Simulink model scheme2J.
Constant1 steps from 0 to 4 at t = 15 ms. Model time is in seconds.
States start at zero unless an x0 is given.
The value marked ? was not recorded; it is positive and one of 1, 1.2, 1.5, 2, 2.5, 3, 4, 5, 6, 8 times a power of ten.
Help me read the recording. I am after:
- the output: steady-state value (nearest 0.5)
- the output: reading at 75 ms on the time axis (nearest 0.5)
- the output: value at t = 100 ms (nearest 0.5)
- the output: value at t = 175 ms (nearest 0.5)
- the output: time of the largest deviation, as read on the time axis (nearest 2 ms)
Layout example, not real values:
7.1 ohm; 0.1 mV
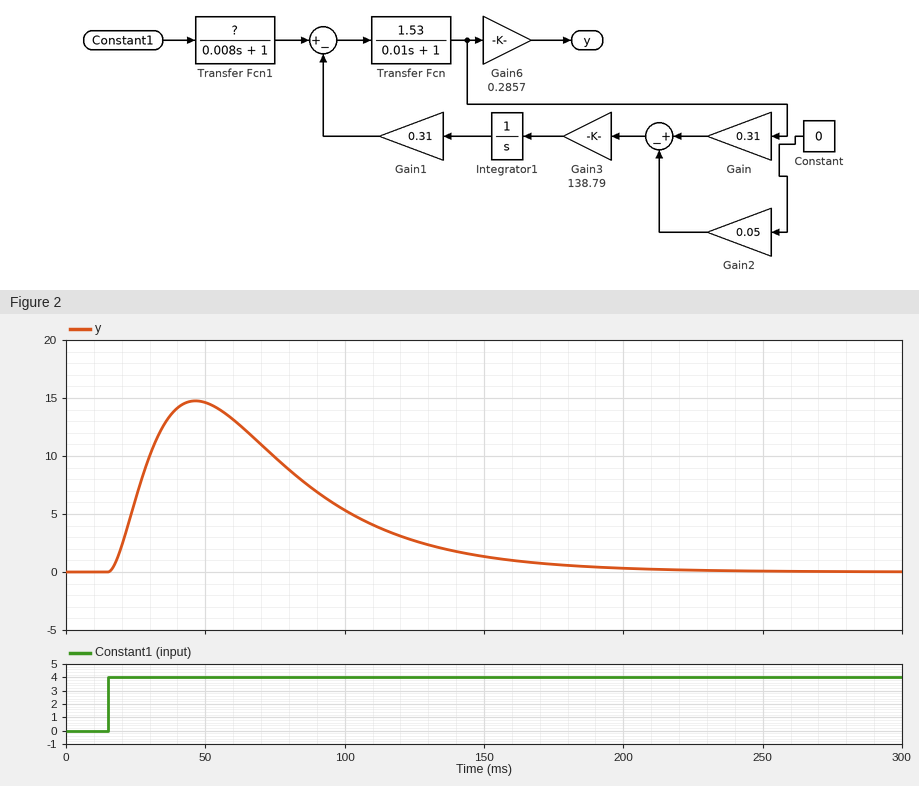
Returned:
0.0; 10.0; 5.5; 0.5; 46 ms
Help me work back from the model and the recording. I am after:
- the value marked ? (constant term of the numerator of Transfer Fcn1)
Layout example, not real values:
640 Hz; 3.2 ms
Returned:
12
